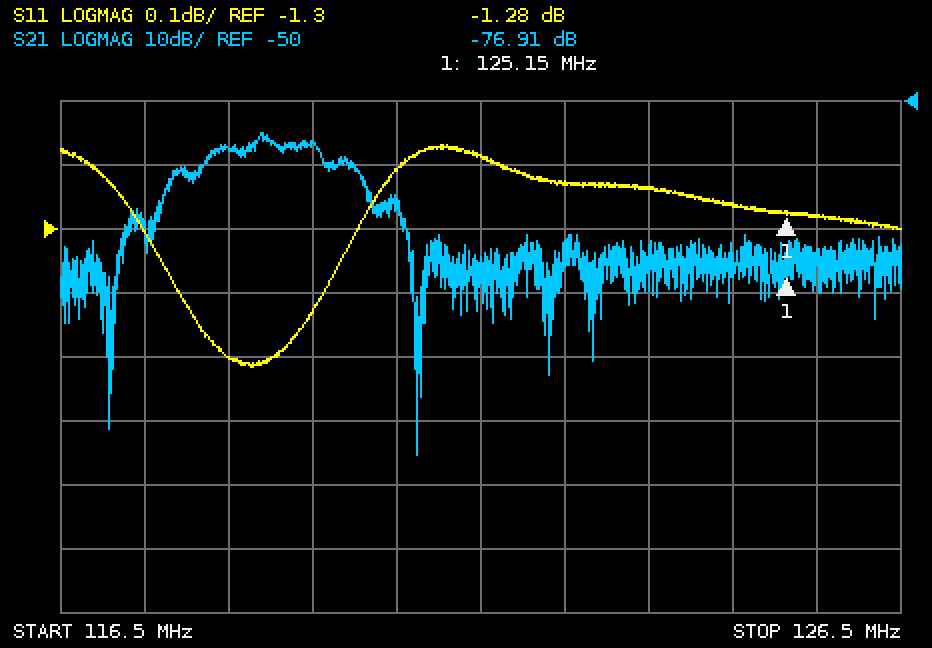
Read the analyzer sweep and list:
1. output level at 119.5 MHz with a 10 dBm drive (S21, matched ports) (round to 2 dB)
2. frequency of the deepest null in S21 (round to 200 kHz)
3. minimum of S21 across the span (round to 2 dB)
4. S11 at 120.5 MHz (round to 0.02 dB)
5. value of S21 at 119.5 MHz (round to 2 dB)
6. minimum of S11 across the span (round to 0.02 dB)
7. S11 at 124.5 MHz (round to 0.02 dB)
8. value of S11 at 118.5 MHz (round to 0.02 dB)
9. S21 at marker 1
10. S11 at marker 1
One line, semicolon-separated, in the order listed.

-46 dBm; 120.8 MHz; -106 dB; -1.20 dB; -56 dB; -1.52 dB; -1.26 dB; -1.50 dB; -76.91 dB; -1.28 dB
